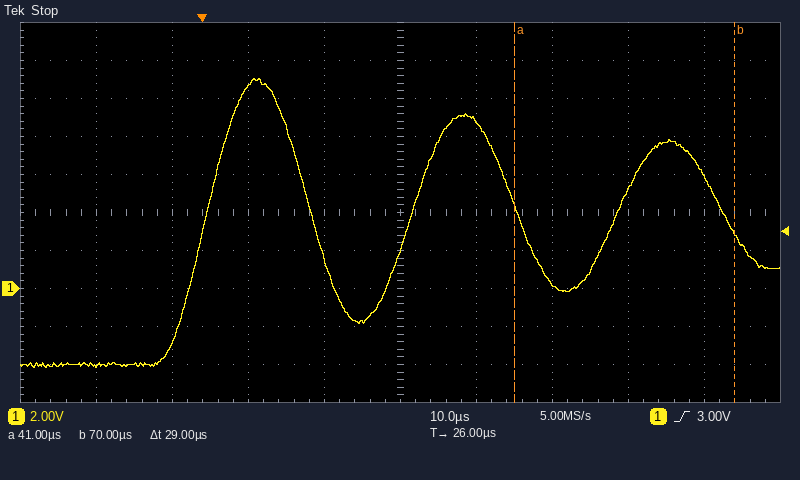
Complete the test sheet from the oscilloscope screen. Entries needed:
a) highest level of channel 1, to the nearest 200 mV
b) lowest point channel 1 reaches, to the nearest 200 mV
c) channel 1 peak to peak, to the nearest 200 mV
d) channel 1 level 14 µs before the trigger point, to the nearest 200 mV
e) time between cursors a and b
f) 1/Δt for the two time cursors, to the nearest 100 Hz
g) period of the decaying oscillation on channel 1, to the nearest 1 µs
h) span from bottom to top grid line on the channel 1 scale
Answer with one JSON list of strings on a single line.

["11.0 V", "-4.2 V", "15.2 V", "-4.0 V", "29 µs", "34.5 kHz", "27 µs", "20 V"]
